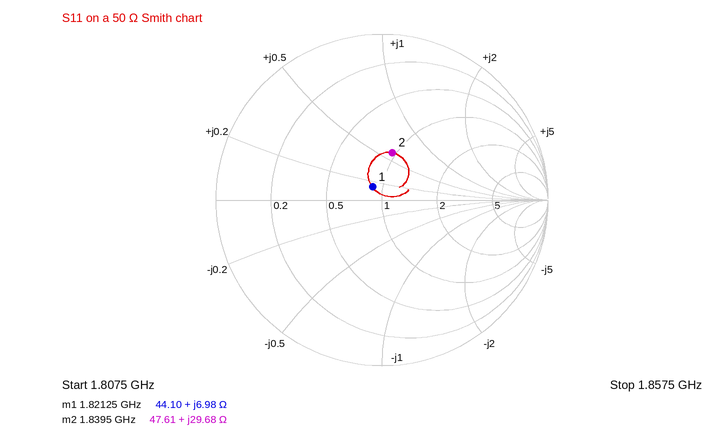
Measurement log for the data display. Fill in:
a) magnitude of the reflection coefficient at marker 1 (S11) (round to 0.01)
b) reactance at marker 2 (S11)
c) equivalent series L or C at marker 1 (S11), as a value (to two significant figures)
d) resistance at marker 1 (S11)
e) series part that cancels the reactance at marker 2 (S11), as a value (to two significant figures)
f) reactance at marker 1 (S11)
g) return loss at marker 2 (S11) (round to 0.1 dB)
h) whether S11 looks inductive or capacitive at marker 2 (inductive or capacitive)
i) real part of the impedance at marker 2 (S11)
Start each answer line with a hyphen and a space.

- 0.10
- +29.68 Ω
- 610 pH
- 44.10 Ω
- 2.9 pF
- +6.98 Ω
- 10.7 dB
- inductive
- 47.61 Ω
